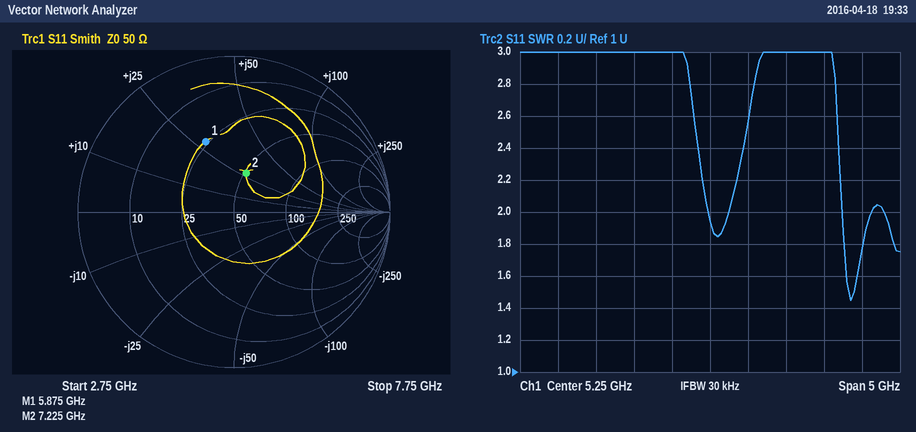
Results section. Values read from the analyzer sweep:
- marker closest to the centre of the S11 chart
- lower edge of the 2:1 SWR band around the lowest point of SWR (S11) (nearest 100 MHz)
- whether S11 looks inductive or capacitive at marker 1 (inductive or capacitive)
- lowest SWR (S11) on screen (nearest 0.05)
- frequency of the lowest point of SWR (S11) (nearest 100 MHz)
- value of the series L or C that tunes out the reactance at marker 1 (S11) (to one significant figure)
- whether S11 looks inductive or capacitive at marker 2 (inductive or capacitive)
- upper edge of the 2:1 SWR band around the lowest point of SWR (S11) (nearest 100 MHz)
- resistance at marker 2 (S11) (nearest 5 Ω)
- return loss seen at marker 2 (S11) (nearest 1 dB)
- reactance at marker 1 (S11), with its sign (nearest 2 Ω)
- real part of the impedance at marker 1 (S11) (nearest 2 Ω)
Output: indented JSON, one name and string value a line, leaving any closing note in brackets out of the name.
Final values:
{
  "marker closest to the centre of the S11 chart": "marker 2",
  "lower edge of the 2:1 SWR band around the lowest point of SWR (S11)": "7.0 GHz",
  "whether S11 looks inductive or capacitive at marker 1": "inductive",
  "lowest SWR (S11) on screen": "1.45",
  "frequency of the lowest point of SWR (S11)": "7.1 GHz",
  "value of the series L or C that tunes out the reactance at marker 1 (S11)": "1.0 pF",
  "whether S11 looks inductive or capacitive at marker 2": "inductive",
  "upper edge of the 2:1 SWR band around the lowest point of SWR (S11)": "7.4 GHz",
  "resistance at marker 2 (S11)": "50 Ω",
  "return loss seen at marker 2 (S11)": "12 dB",
  "reactance at marker 1 (S11), with its sign": "+28 Ω",
  "real part of the impedance at marker 1 (S11)": "24 Ω"
}
